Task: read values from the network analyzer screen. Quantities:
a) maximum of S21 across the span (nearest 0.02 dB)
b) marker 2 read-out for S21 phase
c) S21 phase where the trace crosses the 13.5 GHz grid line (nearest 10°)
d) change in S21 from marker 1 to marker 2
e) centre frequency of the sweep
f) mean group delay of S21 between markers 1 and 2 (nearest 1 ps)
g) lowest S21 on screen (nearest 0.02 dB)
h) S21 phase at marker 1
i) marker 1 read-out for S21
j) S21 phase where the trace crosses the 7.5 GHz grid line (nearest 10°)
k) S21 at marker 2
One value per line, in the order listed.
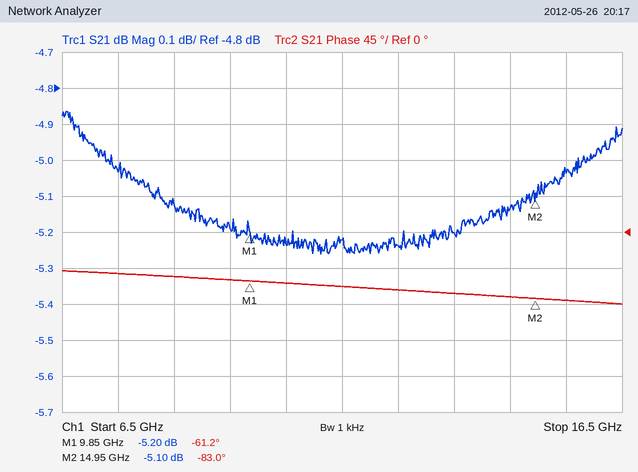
-4.86 dB
-83.0°
-80°
0.10 dB
11.5 GHz
12 ps
-5.26 dB
-61.2°
-5.20 dB
-50°
-5.10 dB
